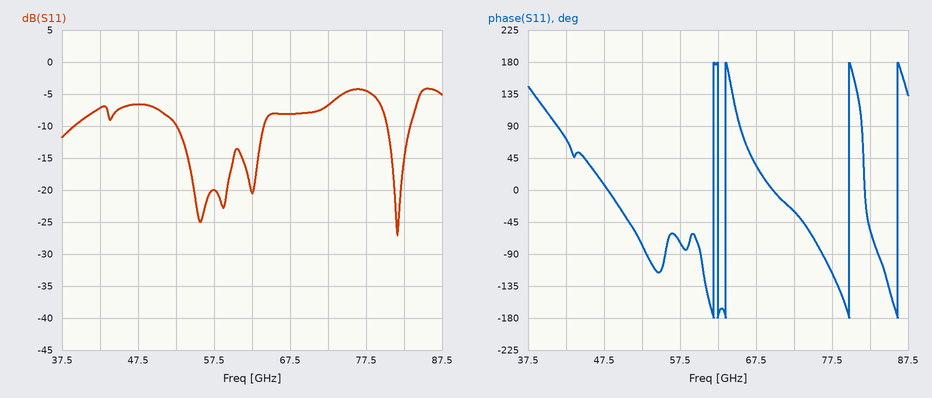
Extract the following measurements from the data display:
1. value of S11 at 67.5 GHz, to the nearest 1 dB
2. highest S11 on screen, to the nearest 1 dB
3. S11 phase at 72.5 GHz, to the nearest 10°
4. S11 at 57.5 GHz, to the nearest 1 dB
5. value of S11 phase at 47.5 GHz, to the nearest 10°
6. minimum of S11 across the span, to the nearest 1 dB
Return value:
-8 dB
-4 dB
-30°
-20 dB
10°
-27 dB
